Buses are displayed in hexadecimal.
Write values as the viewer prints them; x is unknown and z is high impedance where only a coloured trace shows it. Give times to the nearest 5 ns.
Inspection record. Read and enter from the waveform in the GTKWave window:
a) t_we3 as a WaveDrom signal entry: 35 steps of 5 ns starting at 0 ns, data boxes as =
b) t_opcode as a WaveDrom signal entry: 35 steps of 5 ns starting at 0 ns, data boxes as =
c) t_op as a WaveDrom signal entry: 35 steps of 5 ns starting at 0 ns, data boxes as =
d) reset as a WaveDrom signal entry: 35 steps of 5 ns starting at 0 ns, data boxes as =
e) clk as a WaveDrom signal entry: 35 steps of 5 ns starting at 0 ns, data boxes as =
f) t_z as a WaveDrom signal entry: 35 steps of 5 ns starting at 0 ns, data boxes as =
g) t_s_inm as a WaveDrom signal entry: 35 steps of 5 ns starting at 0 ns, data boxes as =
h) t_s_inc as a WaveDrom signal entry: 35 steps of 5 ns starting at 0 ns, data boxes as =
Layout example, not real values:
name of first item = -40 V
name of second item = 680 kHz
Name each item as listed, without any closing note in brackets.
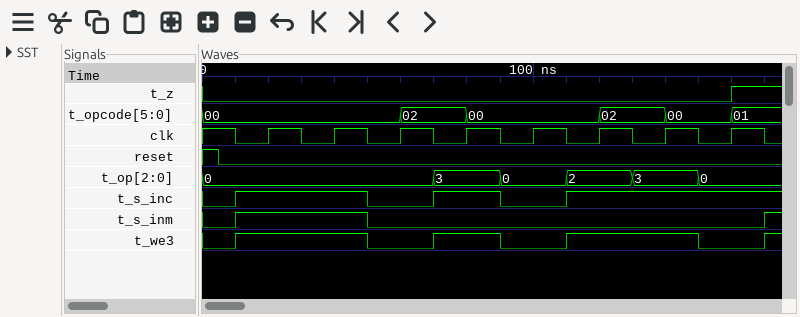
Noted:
t_we3 as a WaveDrom signal entry: 35 steps of 5 ns starting at 0 ns, data boxes as = = {name: 't_we3', wave: '0.1.......0...1...0...1.......0...1'}
t_opcode as a WaveDrom signal entry: 35 steps of 5 ns starting at 0 ns, data boxes as = = {name: 't_opcode', wave: '=...........=...=.......=...=...=..', data: '00 02 00 02 00 01'}
t_op as a WaveDrom signal entry: 35 steps of 5 ns starting at 0 ns, data boxes as = = {name: 't_op', wave: '=.............=...=...=...=...=....', data: '0 3 0 2 3 0'}
reset as a WaveDrom signal entry: 35 steps of 5 ns starting at 0 ns, data boxes as = = {name: 'reset', wave: '10.................................'}
clk as a WaveDrom signal entry: 35 steps of 5 ns starting at 0 ns, data boxes as = = {name: 'clk', wave: '1.0.1.0.1.0.1.0.1.0.1.0.1.0.1.0.1.0'}
t_z as a WaveDrom signal entry: 35 steps of 5 ns starting at 0 ns, data boxes as = = {name: 't_z', wave: '0...............................1..'}
t_s_inm as a WaveDrom signal entry: 35 steps of 5 ns starting at 0 ns, data boxes as = = {name: 't_s_inm', wave: '0.1.......0.......................1'}
t_s_inc as a WaveDrom signal entry: 35 steps of 5 ns starting at 0 ns, data boxes as = = {name: 't_s_inc', wave: '0.1.......0...1...0...1............'}
